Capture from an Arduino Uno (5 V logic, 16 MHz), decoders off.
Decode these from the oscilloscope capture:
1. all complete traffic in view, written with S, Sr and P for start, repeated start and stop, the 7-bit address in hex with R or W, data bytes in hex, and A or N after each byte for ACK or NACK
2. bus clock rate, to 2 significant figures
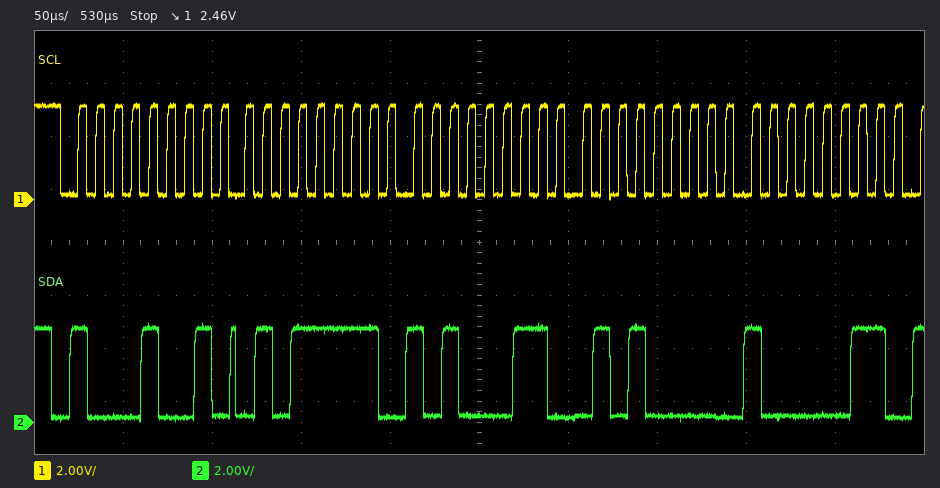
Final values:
S 44R A 5F A A3 A 50 A 83 A
100 kHz
